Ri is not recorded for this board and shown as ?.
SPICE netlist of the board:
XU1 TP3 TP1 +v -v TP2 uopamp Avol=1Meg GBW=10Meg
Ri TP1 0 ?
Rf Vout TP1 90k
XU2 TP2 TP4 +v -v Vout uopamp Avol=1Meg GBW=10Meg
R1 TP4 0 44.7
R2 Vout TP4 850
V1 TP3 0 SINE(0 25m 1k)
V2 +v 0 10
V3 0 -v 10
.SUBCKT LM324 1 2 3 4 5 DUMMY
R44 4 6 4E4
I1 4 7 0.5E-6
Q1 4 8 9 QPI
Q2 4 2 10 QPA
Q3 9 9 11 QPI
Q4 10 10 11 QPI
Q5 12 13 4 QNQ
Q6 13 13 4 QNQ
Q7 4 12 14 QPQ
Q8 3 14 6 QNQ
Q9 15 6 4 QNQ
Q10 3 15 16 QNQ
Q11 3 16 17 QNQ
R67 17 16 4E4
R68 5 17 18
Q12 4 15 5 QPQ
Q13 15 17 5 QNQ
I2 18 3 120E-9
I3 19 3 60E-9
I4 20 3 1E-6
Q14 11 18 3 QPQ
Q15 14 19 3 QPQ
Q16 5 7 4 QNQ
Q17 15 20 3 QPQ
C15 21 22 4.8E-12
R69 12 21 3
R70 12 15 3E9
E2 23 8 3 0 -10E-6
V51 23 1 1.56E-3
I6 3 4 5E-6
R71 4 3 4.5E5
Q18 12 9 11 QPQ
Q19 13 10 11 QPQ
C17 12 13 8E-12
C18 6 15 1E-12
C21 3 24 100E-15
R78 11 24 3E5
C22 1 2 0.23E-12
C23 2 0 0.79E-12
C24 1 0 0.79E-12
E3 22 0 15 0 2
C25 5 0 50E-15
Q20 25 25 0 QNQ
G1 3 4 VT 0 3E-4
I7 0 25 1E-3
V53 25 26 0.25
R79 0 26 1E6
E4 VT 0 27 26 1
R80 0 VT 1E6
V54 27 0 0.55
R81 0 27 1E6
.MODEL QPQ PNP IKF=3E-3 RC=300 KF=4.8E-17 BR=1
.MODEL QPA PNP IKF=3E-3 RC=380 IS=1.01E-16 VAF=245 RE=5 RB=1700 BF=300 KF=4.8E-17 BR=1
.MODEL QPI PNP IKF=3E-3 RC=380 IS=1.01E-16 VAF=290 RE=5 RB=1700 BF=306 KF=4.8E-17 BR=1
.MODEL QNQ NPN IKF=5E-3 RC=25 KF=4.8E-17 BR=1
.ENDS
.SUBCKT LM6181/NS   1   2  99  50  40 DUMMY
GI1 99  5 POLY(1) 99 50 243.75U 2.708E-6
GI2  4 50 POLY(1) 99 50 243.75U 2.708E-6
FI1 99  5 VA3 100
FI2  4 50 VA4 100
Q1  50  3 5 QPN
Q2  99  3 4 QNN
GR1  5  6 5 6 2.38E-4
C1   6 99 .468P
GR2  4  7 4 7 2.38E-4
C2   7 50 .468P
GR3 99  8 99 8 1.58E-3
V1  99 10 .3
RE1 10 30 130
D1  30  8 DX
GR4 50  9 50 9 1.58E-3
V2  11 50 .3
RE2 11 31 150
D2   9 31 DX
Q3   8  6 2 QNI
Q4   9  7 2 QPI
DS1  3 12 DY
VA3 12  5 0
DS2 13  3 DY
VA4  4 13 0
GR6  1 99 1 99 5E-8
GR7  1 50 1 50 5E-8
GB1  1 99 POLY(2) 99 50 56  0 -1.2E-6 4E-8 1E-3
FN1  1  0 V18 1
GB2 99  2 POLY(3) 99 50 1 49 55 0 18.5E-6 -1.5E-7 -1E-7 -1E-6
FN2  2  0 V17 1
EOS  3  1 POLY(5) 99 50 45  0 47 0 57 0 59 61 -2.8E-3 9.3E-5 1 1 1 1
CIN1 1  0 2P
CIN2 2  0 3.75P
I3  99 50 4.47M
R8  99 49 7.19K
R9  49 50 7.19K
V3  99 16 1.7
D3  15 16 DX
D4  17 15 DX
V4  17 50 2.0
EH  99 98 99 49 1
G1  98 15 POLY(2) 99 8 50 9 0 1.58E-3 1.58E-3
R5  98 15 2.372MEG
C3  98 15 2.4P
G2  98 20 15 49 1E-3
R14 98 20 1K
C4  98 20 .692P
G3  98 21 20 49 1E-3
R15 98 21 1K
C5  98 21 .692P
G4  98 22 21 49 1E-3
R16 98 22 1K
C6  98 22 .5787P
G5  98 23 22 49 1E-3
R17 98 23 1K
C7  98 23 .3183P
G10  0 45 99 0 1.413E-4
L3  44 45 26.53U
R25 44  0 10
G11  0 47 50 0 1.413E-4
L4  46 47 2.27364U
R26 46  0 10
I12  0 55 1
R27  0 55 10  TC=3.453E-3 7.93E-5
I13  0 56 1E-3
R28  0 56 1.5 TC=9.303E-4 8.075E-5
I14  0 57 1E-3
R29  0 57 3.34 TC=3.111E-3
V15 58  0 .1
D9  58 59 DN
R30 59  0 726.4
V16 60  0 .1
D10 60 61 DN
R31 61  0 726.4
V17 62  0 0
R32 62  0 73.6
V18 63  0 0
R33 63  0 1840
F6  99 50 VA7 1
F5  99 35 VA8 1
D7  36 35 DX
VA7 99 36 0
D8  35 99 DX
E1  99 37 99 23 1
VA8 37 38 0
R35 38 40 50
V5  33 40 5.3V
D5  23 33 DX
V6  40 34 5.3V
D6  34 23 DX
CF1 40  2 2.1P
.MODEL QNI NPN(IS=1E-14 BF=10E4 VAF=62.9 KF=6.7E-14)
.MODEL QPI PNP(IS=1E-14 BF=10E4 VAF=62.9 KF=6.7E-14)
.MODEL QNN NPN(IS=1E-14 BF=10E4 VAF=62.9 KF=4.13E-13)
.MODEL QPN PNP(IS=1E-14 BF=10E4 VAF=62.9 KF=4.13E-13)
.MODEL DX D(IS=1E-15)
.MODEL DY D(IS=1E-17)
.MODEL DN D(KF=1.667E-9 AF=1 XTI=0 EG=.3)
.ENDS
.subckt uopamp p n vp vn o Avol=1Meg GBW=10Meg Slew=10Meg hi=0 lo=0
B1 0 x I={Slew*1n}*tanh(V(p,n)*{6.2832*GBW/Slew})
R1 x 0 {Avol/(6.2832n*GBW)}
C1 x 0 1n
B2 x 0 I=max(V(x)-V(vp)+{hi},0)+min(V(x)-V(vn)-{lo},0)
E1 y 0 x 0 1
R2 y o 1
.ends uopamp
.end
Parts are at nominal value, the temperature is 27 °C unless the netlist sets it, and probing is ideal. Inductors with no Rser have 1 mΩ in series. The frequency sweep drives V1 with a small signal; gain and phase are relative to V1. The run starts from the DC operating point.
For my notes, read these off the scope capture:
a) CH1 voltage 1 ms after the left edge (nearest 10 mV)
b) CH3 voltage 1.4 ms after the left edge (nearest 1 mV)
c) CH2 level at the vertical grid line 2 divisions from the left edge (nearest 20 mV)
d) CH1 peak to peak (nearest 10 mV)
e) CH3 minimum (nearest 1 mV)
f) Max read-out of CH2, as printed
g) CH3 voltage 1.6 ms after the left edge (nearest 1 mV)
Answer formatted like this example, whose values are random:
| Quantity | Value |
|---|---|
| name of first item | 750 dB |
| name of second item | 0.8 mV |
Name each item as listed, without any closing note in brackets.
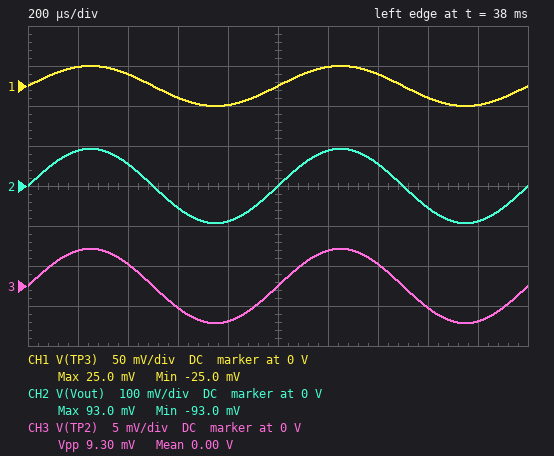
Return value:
| Quantity | Value |
|---|---|
| CH1 voltage 1 ms after the left edge | 0 V |
| CH3 voltage 1.4 ms after the left edge | 3 mV |
| CH2 level at the vertical grid line 2 divisions from the left edge | 60 mV |
| CH1 peak to peak | 50 mV |
| CH3 minimum | -5 mV |
| Max read-out of CH2, as printed | 93.0 mV |
| CH3 voltage 1.6 ms after the left edge | -3 mV |
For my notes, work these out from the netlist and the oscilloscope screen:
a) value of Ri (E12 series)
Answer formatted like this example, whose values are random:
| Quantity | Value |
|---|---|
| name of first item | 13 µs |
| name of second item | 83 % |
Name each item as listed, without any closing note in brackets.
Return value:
| Quantity | Value |
|---|---|
| value of Ri | 33 kΩ |
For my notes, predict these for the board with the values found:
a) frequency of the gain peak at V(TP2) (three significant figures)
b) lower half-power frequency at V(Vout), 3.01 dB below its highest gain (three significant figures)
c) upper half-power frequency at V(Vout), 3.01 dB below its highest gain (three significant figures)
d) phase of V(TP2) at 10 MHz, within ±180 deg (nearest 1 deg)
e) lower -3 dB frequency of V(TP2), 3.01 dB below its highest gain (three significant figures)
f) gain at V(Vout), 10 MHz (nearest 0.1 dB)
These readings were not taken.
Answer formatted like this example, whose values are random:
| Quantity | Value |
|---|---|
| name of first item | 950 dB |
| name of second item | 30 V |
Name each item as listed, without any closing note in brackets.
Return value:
| Quantity | Value |
|---|---|
| frequency of the gain peak at V(TP2) | 5.18 MHz |
| lower half-power frequency at V(Vout), 3.01 dB below its highest gain | 4.91 MHz |
| upper half-power frequency at V(Vout), 3.01 dB below its highest gain | 5.41 MHz |
| phase of V(TP2) at 10 MHz, within ±180 deg | -89 deg |
| lower -3 dB frequency of V(TP2), 3.01 dB below its highest gain | 4.93 MHz |
| gain at V(Vout), 10 MHz | 2.7 dB |
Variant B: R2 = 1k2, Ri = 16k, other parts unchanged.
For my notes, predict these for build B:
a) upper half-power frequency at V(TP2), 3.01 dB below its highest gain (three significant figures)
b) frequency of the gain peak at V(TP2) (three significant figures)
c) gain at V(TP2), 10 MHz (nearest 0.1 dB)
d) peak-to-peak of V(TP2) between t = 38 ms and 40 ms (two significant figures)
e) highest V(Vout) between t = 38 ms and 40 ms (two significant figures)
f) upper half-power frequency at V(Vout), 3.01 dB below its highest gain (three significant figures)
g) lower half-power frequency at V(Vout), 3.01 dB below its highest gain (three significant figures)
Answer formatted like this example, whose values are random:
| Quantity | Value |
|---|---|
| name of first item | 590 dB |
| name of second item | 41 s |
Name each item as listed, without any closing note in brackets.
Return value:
| Quantity | Value |
|---|---|
| upper half-power frequency at V(TP2), 3.01 dB below its highest gain | 4.07 MHz |
| frequency of the gain peak at V(TP2) | 3.88 MHz |
| gain at V(TP2), 10 MHz | 1.4 dB |
| peak-to-peak of V(TP2) between t = 38 ms and 40 ms | 12 mV |
| highest V(Vout) between t = 38 ms and 40 ms | 170 mV |
| upper half-power frequency at V(Vout), 3.01 dB below its highest gain | 4.05 MHz |
| lower half-power frequency at V(Vout), 3.01 dB below its highest gain | 3.69 MHz |
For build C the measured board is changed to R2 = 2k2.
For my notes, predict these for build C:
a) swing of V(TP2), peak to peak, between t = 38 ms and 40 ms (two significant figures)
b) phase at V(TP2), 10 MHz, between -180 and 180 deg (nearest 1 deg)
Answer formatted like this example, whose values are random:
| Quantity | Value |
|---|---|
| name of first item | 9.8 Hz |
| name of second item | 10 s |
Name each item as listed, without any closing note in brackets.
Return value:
| Quantity | Value |
|---|---|
| swing of V(TP2), peak to peak, between t = 38 ms and 40 ms | 3.7 mV |
| phase at V(TP2), 10 MHz, between -180 and 180 deg | -90 deg |
